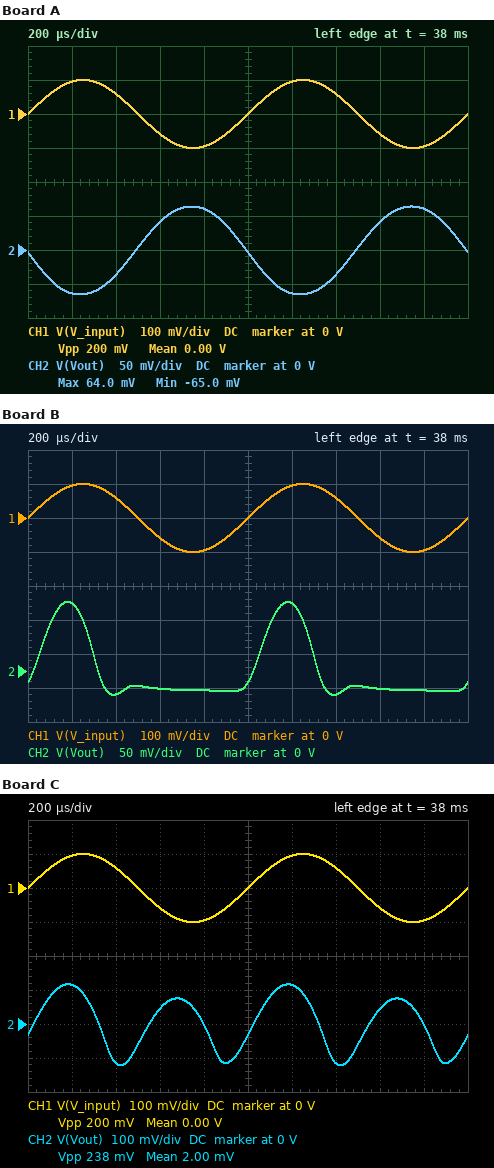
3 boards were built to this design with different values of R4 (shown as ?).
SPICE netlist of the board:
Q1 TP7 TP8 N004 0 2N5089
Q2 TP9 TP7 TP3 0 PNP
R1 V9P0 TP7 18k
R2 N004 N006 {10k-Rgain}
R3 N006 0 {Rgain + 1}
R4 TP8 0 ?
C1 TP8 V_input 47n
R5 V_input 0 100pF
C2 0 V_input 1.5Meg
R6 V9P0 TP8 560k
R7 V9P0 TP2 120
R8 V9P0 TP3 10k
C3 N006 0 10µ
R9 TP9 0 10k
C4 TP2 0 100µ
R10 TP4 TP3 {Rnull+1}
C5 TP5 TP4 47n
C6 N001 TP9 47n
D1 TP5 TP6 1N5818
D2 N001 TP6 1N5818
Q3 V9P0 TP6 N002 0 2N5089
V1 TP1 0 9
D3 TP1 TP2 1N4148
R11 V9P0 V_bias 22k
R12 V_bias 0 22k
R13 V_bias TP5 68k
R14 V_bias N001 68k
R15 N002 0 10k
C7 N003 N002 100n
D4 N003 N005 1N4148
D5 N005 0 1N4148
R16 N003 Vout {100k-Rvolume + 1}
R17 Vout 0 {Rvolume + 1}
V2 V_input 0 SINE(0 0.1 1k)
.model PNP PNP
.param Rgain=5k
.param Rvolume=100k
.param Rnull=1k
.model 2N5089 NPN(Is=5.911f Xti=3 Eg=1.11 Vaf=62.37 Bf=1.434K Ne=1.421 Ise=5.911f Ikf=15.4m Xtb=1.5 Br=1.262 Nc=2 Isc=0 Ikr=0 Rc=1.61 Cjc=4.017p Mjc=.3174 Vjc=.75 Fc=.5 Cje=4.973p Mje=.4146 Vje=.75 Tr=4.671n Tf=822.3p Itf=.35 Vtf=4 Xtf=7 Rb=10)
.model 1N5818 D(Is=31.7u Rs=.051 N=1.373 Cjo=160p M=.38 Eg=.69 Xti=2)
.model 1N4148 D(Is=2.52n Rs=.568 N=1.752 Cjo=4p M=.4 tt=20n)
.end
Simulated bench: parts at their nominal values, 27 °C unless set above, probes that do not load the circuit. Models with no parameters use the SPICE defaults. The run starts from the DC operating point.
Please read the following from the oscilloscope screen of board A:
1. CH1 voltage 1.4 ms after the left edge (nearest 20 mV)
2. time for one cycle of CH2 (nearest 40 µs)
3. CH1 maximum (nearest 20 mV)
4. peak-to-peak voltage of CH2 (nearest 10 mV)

60 mV
1.00 ms
100 mV
130 mV
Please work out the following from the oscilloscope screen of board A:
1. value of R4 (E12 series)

470 kΩ
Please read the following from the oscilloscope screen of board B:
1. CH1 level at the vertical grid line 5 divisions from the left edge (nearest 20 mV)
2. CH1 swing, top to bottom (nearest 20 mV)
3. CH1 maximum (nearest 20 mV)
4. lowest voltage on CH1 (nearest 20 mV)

0 V
200 mV
100 mV
-100 mV
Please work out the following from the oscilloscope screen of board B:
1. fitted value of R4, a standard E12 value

82 kΩ
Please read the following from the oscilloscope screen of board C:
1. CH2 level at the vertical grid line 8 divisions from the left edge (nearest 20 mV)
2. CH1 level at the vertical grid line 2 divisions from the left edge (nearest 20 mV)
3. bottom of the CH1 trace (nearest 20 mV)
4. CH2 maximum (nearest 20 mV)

40 mV
60 mV
-100 mV
120 mV
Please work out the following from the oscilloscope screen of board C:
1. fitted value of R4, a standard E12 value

120 kΩ
